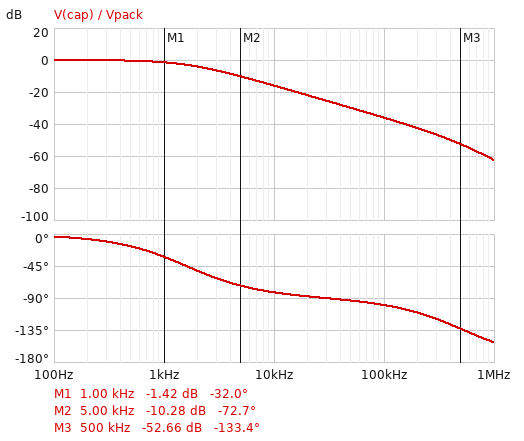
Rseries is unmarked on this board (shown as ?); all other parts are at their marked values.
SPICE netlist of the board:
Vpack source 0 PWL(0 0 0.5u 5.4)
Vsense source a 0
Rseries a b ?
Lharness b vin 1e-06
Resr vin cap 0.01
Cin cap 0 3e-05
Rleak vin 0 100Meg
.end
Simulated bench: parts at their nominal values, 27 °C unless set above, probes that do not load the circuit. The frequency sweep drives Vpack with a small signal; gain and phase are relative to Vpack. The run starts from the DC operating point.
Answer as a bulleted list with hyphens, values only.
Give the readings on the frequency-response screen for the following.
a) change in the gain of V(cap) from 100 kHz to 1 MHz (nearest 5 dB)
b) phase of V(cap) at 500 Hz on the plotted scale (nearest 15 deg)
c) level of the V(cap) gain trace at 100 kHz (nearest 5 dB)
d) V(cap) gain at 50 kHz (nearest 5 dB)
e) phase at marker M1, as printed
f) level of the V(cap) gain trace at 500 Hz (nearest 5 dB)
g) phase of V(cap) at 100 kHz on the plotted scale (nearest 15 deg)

- -25 dB
- -15 deg
- -35 dB
- -30 dB
- -32.0 deg
- 0 dB
- -105 deg
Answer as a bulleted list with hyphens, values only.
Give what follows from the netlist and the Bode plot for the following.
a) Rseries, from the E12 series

- 3.3 Ω
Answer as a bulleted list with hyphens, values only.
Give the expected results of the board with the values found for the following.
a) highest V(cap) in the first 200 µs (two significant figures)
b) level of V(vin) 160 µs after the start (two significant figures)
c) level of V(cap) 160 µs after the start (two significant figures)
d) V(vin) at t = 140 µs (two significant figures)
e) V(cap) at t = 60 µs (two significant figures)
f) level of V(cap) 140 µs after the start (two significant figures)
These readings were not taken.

- 4.7 V
- 4.3 V
- 4.3 V
- 4.1 V
- 2.4 V
- 4.1 V
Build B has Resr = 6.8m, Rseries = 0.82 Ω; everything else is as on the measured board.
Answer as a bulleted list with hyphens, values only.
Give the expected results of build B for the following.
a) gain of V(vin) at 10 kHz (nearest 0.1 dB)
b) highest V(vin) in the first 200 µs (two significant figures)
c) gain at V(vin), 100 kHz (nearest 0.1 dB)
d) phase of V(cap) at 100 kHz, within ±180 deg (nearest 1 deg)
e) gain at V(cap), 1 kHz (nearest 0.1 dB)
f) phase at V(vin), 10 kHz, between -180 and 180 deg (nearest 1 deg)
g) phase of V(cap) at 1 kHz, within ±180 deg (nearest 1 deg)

- -5.1 dB
- 5.4 V
- -25.5 dB
- -125 deg
- -0.1 dB
- -60 deg
- -9 deg
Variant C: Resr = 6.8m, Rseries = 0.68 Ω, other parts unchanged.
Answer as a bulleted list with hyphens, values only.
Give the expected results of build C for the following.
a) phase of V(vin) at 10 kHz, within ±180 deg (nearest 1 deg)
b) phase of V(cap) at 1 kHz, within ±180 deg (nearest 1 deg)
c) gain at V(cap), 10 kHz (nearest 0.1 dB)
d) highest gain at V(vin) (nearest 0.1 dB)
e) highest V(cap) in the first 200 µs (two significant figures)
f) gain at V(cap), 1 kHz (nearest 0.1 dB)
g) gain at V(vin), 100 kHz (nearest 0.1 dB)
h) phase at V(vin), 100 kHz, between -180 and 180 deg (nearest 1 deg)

- -55 deg
- -7 deg
- -3.9 dB
- 0 dB
- 5.4 V
- -0.1 dB
- -24.5 dB
- -123 deg
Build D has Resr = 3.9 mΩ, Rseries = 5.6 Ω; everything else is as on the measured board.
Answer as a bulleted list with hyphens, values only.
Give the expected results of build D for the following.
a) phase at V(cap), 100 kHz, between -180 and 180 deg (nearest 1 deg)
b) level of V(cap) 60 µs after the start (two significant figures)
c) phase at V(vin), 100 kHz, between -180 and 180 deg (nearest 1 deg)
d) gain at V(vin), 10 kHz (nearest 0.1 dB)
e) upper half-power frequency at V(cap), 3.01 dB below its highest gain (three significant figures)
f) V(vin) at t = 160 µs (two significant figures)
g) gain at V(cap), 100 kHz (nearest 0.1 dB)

- -96 deg
- 1.6 V
- -92 deg
- -20.5 dB
- 948 Hz
- 3.3 V
- -40.5 dB
